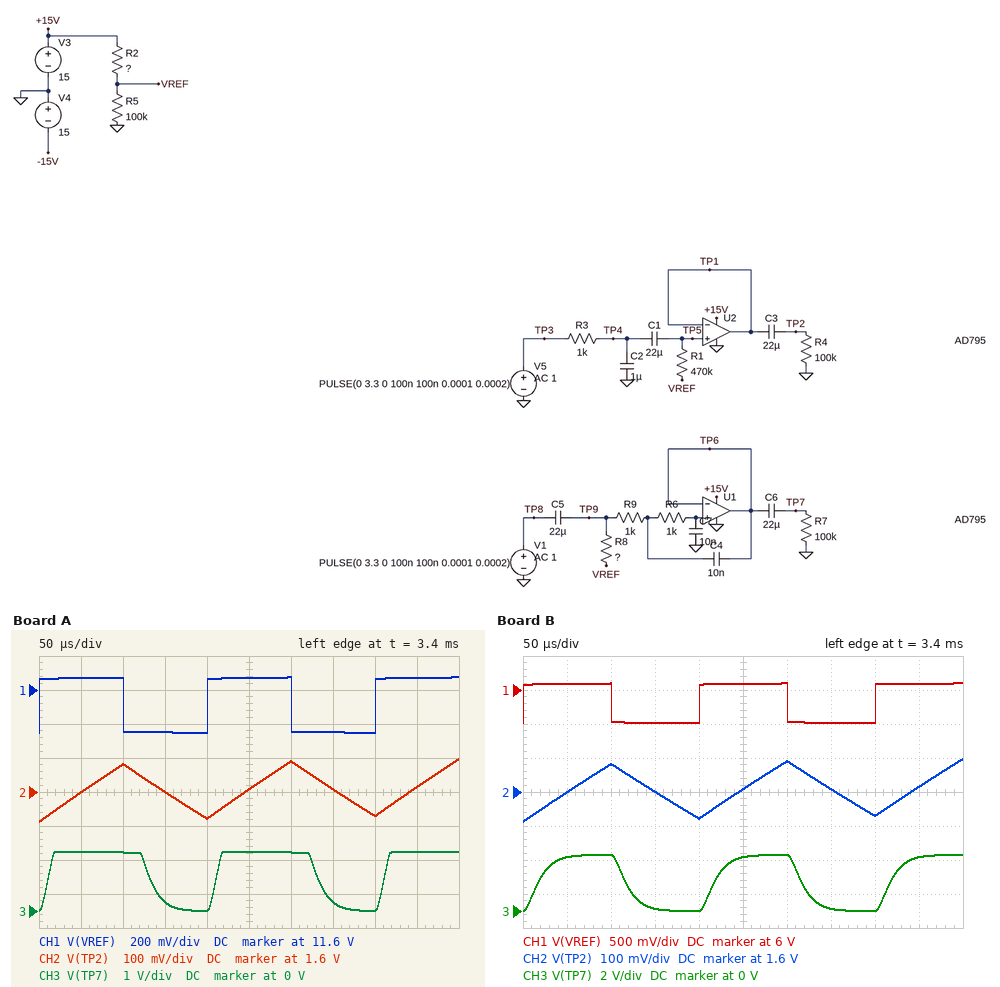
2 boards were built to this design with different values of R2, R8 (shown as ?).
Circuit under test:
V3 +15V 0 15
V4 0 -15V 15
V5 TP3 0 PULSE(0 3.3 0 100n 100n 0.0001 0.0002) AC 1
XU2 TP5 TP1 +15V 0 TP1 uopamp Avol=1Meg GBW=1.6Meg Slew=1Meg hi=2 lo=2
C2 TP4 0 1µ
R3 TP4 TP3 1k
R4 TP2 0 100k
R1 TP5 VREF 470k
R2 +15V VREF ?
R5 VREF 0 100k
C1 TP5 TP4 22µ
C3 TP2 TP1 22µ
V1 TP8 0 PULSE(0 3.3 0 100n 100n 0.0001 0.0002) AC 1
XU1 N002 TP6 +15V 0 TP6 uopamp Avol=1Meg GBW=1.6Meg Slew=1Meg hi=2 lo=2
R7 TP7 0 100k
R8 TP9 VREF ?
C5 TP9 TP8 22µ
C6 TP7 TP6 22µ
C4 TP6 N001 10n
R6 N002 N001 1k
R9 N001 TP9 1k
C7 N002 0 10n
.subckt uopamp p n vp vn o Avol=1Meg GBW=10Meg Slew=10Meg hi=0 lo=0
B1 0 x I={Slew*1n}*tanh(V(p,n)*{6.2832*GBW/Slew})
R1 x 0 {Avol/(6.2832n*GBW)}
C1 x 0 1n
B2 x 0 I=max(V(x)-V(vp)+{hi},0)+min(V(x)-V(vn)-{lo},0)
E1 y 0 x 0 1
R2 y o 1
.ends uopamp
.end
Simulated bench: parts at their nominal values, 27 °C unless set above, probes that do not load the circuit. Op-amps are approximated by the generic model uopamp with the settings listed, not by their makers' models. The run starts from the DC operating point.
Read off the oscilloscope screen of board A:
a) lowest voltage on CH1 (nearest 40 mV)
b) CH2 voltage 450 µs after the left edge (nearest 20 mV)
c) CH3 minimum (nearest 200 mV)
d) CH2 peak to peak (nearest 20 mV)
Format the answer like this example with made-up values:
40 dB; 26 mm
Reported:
11.36 V; 1.62 V; 0 V; 180 mV
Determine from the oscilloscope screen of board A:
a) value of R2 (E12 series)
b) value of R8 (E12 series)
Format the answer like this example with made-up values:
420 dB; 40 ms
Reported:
33 kΩ; 220 kΩ
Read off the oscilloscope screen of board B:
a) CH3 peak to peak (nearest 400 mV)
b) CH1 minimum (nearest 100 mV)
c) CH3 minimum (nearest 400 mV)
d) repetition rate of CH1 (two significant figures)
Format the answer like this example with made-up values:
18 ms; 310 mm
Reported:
3.2 V; 5.5 V; 0 V; 5.0 kHz
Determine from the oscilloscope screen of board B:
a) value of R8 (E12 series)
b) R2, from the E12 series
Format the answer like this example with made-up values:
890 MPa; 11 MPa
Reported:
270 kΩ; 180 kΩ
